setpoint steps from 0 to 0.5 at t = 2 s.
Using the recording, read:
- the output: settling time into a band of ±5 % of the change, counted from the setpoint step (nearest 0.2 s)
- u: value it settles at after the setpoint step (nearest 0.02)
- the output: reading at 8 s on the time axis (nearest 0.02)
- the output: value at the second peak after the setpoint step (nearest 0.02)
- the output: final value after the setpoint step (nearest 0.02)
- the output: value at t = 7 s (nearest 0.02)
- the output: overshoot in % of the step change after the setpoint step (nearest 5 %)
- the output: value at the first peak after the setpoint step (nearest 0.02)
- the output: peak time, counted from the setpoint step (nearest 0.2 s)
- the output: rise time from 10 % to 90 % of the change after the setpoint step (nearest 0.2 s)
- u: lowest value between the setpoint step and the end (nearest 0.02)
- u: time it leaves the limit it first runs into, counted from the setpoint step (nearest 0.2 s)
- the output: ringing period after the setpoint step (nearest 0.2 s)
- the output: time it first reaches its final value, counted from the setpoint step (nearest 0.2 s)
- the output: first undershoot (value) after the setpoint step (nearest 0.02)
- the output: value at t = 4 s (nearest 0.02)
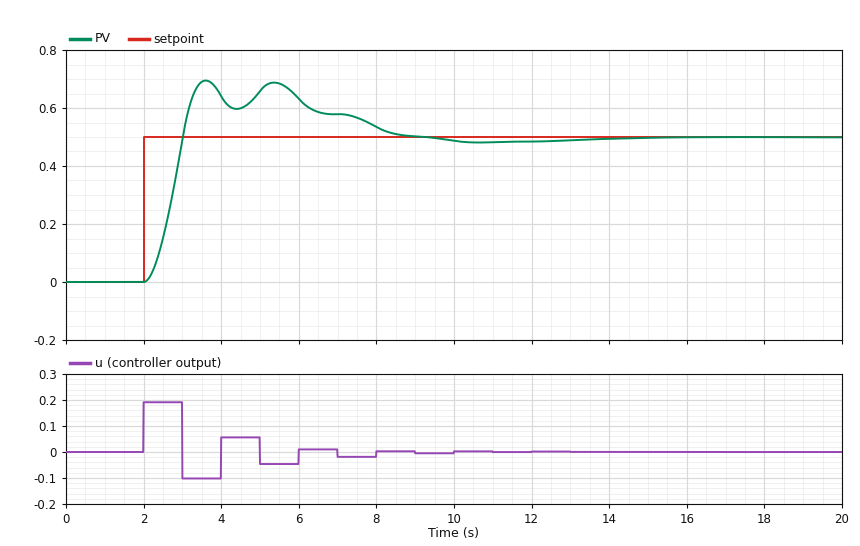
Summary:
6.2 s
0.00
0.54
0.68
0.50
0.58
40 %
0.70
1.6 s
0.6 s
-0.10
1.0 s
1.8 s
1.0 s
0.60
0.64
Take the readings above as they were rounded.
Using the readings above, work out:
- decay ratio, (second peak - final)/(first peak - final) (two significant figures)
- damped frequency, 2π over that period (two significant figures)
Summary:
0.90
3.5 rad/s
